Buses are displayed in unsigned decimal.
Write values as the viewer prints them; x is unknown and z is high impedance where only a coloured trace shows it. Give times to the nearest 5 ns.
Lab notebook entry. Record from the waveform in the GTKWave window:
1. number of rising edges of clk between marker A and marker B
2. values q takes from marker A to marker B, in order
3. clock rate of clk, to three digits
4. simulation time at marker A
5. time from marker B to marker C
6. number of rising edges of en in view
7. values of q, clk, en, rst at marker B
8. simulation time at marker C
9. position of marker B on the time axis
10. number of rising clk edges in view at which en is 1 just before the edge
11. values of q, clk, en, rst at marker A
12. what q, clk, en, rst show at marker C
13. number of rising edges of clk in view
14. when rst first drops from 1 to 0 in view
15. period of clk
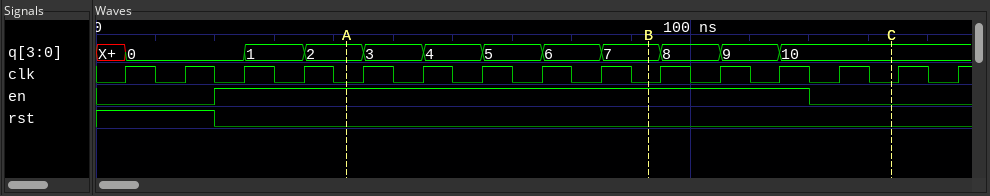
5
2, 3, 4, 5, 6, 7
100 MHz
40 ns
40 ns
1
q=7, clk=0, en=1, rst=0
135 ns
95 ns
10
q=2, clk=0, en=1, rst=0
q=10, clk=0, en=0, rst=0
15
20 ns
10 ns
